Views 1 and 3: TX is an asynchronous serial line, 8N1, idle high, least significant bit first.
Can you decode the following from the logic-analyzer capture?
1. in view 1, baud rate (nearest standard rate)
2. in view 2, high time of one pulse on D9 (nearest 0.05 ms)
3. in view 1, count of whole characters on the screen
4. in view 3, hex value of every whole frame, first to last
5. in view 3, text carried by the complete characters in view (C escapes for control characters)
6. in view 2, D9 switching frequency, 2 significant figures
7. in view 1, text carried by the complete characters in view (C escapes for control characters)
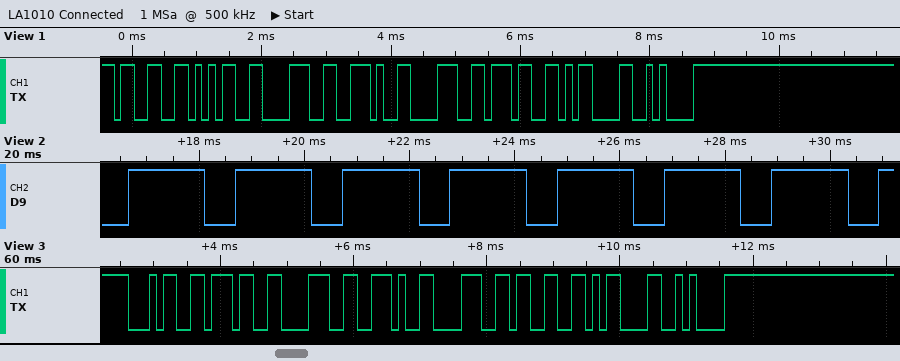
9600 baud
1.45 ms
8
34 37 38 2E 38 33 0D 0A
"478.83\r\n"
490 Hz
"358.87\r\n"
